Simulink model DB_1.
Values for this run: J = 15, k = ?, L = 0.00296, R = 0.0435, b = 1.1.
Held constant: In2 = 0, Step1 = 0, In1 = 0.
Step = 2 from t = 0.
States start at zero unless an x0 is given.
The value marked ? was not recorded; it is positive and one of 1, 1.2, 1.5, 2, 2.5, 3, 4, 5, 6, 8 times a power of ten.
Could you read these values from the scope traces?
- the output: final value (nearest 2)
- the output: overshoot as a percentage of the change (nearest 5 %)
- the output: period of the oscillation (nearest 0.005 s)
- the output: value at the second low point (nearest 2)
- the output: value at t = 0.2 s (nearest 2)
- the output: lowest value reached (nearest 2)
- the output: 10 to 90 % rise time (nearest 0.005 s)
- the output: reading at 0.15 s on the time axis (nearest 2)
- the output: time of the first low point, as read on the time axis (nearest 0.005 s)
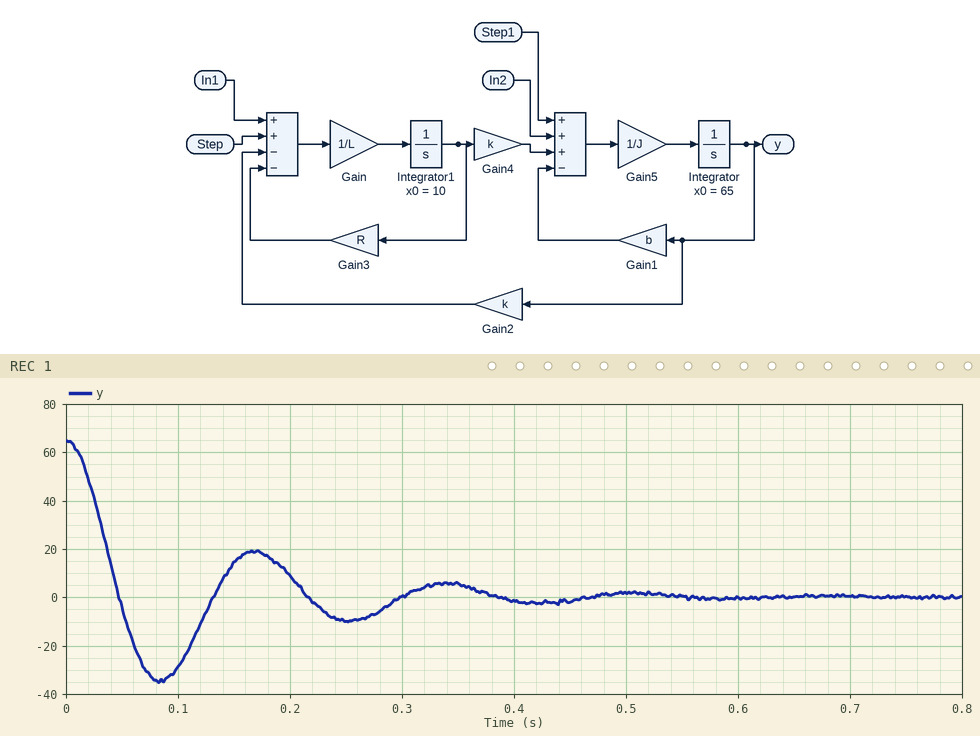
0
55 %
0.170 s
-10
8
-34
0.030 s
14
0.085 s
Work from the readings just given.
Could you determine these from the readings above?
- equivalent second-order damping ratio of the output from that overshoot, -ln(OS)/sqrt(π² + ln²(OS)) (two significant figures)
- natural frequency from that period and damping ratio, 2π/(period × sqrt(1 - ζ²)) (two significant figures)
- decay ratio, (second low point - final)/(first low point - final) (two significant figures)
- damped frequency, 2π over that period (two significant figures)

0.19
38 rad/s
0.29
37 rad/s
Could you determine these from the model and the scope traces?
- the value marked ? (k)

8
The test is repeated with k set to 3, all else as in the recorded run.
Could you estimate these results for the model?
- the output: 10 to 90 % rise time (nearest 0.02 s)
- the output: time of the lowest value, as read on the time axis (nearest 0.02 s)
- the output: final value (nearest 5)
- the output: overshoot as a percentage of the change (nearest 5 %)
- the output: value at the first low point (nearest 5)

0.12 s
0.26 s
0
15 %
-10
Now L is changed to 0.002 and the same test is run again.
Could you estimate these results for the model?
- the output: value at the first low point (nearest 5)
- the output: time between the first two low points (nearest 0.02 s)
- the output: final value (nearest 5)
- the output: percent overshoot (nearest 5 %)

-30
0.14 s
0
45 %
